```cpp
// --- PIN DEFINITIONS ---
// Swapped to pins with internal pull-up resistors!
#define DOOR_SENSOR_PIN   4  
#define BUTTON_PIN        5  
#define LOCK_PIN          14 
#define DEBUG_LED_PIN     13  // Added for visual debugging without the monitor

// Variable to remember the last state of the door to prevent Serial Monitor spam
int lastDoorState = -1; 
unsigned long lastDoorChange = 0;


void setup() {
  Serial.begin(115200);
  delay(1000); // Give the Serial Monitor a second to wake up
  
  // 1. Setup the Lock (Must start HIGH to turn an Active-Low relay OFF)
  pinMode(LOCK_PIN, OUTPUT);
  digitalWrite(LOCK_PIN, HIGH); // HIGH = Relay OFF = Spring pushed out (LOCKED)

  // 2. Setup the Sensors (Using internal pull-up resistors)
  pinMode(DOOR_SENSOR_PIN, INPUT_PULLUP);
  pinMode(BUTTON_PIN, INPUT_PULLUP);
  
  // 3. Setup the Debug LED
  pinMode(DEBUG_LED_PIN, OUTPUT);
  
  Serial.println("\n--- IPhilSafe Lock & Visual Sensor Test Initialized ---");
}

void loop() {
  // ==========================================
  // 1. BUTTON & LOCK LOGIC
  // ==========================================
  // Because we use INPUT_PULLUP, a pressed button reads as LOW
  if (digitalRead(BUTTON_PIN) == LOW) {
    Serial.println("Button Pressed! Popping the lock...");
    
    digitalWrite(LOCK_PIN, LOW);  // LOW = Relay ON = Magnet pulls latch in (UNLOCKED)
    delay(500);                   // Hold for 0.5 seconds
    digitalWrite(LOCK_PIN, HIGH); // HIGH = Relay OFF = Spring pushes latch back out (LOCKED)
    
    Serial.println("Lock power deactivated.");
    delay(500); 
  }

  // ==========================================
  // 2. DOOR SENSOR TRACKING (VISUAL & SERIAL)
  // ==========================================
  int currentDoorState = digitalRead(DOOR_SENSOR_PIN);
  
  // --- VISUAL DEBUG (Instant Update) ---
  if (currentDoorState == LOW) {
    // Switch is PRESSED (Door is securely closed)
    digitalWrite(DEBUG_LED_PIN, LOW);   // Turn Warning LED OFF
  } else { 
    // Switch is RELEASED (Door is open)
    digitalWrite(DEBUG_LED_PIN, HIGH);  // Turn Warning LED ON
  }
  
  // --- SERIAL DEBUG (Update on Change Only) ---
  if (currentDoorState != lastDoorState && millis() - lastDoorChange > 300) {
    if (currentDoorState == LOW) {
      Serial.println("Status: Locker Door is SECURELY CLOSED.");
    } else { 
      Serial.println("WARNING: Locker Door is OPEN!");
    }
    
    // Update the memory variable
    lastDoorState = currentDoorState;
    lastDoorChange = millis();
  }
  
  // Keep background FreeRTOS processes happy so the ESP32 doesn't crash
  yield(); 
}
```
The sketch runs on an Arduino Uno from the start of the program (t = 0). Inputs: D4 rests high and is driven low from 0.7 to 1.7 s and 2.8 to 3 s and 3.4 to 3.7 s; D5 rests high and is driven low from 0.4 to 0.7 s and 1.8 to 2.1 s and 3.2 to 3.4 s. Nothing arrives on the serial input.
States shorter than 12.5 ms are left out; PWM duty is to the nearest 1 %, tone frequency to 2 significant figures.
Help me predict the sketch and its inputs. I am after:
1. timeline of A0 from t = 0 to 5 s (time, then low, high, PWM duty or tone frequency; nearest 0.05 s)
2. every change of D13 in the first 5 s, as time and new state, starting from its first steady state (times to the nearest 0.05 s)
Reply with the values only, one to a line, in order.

1 s high; 1.8 s low; 2.3 s high; 3.2 s low; 3.7 s high
1 s low; 1.7 s high; 2.8 s low; 3 s high
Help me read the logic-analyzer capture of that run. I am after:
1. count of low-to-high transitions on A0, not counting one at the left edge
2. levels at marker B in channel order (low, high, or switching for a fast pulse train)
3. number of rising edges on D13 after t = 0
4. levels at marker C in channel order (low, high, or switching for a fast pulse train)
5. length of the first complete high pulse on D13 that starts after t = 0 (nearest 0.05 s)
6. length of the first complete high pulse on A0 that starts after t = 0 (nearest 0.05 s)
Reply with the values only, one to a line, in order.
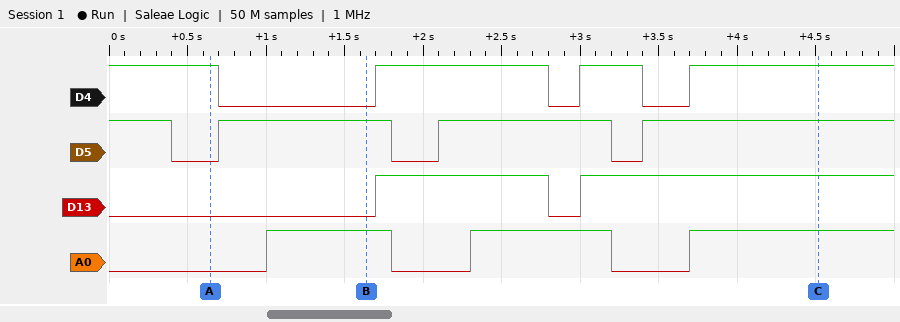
3
D4 low, D5 high, D13 low, A0 high
2
D4 high, D5 high, D13 high, A0 high
1.10 s
0.80 s
